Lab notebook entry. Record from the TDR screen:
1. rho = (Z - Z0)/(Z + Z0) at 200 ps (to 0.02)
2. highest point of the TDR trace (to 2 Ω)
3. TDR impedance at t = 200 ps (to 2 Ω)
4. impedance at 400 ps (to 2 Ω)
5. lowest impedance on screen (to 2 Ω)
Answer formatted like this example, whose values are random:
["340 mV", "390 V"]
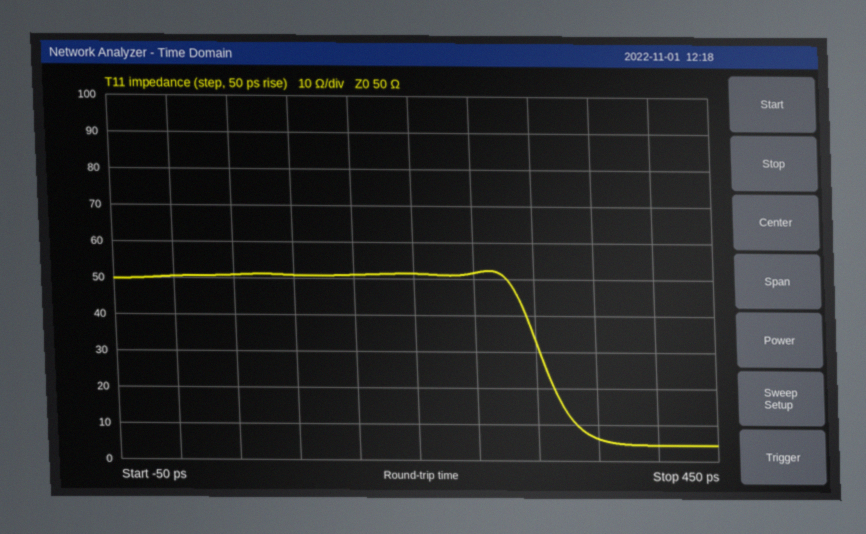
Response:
["+0.02", "52 Ω", "52 Ω", "4 Ω", "4 Ω"]
